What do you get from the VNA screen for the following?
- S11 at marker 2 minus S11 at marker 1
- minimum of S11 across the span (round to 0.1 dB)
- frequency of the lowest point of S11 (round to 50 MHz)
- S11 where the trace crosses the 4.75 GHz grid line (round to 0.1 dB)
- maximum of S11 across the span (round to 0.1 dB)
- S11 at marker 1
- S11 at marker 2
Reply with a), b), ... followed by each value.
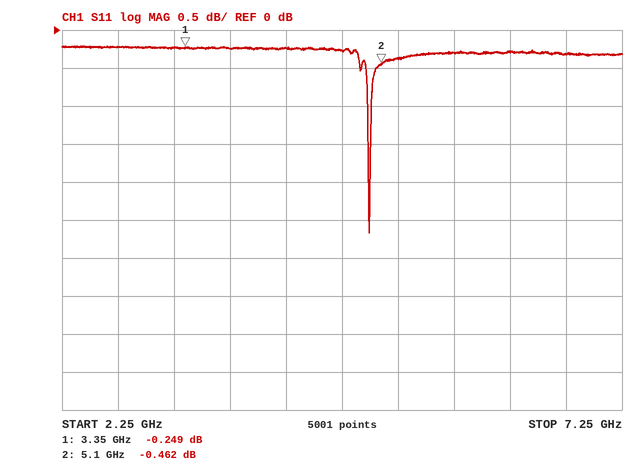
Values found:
a) -0.213 dB
b) -2.7 dB
c) 5.00 GHz
d) -0.3 dB
e) -0.2 dB
f) -0.249 dB
g) -0.462 dB
